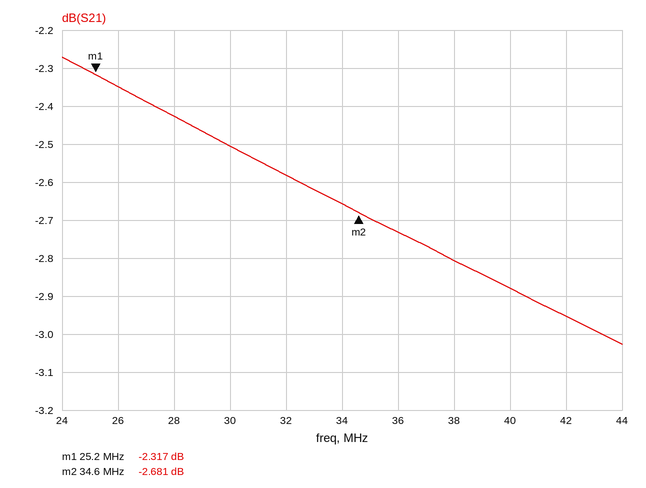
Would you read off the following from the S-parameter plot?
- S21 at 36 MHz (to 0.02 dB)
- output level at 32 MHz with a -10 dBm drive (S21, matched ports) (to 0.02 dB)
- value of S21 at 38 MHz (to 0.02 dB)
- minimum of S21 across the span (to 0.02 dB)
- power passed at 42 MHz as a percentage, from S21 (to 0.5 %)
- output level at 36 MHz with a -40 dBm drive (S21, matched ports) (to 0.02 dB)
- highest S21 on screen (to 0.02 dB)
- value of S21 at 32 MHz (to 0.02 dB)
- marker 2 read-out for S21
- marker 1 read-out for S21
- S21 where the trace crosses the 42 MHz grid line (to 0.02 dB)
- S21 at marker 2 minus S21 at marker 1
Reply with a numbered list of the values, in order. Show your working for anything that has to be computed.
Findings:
1. -2.74 dB
2. -10 dBm + (-2.58 dB) = -12.58 dBm
3. -2.80 dB
4. -3.02 dB
5. 10^(-2.96/10) ≈ 50.6 %, so 50.5 % to the nearest 0.5 %
6. -40 dBm + (-2.74 dB) = -42.74 dBm
7. -2.28 dB
8. -2.58 dB
9. -2.681 dB
10. -2.317 dB
11. -2.96 dB
12. -2.681 − (-2.317) = -0.364 dB
